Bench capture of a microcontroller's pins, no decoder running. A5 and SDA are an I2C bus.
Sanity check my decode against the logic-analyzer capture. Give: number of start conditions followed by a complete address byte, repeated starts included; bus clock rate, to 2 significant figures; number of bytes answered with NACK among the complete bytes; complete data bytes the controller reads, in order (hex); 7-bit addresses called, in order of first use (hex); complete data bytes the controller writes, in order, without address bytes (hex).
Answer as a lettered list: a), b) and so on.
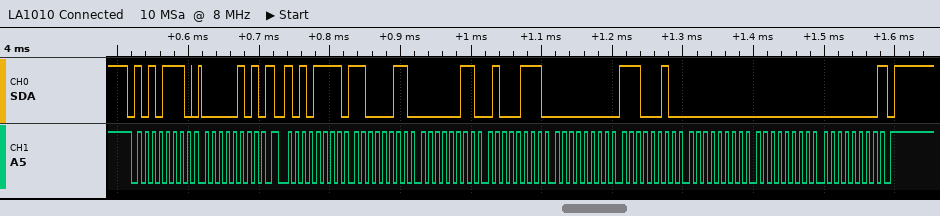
a) 2
b) 100 kHz
c) 1
d) C3 03 47 00 E2 00 00 00
e) 0x57
f) 05
